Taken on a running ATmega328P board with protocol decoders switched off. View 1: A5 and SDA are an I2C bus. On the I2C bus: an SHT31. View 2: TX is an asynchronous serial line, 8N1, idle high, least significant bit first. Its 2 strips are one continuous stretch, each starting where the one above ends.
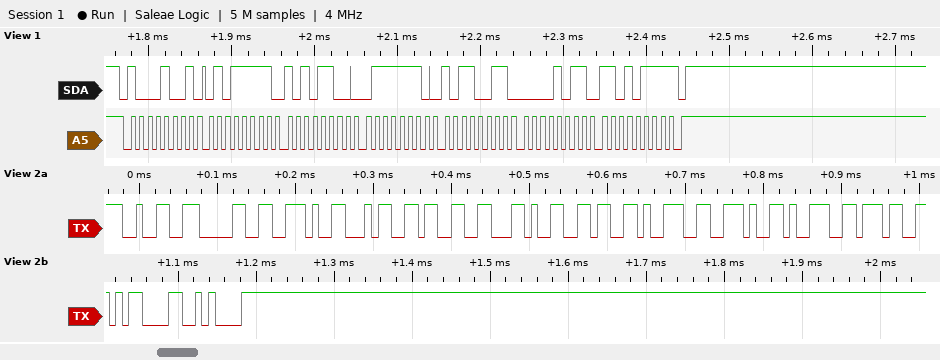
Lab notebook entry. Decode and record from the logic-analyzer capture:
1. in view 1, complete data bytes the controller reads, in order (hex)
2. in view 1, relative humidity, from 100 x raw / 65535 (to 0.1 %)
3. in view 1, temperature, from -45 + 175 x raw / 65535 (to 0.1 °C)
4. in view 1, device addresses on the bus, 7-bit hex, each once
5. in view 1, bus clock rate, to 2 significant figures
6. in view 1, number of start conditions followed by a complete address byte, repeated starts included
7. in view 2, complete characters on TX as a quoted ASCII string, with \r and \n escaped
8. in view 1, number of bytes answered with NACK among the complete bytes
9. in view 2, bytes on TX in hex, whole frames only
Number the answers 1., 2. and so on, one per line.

1. 5F AC 7E B3 0B D7
2. 69.9 %
3. 20.4 °C
4. 0x44
5. 100 kHz
6. 1
7. "20.43,69.97\r\n"
8. 1
9. 32 30 2E 34 33 2C 36 39 2E 39 37 0D 0A
